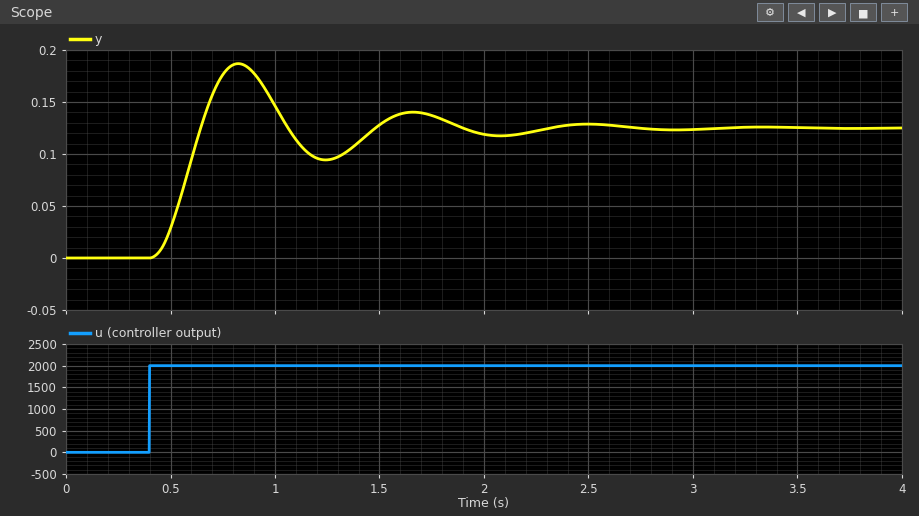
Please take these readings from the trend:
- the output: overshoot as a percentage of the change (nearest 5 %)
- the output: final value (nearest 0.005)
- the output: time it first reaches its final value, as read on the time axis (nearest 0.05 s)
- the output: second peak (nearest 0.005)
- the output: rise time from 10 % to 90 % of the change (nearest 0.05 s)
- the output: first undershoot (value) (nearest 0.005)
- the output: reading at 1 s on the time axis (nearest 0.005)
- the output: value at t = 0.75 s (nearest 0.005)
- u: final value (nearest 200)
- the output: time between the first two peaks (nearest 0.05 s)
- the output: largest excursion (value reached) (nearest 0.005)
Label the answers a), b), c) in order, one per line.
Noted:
a) 50 %
b) 0.125
c) 0.65 s
d) 0.140
e) 0.15 s
f) 0.095
g) 0.145
h) 0.175
i) 2000
j) 0.85 s
k) 0.185
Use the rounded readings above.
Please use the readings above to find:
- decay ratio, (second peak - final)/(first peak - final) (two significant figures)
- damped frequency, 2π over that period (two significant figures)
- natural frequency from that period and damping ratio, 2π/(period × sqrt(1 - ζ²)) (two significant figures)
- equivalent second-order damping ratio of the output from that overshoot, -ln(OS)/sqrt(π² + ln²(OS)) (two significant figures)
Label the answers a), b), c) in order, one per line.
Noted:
a) 0.25
b) 7.4 rad/s
c) 7.6 rad/s
d) 0.22
